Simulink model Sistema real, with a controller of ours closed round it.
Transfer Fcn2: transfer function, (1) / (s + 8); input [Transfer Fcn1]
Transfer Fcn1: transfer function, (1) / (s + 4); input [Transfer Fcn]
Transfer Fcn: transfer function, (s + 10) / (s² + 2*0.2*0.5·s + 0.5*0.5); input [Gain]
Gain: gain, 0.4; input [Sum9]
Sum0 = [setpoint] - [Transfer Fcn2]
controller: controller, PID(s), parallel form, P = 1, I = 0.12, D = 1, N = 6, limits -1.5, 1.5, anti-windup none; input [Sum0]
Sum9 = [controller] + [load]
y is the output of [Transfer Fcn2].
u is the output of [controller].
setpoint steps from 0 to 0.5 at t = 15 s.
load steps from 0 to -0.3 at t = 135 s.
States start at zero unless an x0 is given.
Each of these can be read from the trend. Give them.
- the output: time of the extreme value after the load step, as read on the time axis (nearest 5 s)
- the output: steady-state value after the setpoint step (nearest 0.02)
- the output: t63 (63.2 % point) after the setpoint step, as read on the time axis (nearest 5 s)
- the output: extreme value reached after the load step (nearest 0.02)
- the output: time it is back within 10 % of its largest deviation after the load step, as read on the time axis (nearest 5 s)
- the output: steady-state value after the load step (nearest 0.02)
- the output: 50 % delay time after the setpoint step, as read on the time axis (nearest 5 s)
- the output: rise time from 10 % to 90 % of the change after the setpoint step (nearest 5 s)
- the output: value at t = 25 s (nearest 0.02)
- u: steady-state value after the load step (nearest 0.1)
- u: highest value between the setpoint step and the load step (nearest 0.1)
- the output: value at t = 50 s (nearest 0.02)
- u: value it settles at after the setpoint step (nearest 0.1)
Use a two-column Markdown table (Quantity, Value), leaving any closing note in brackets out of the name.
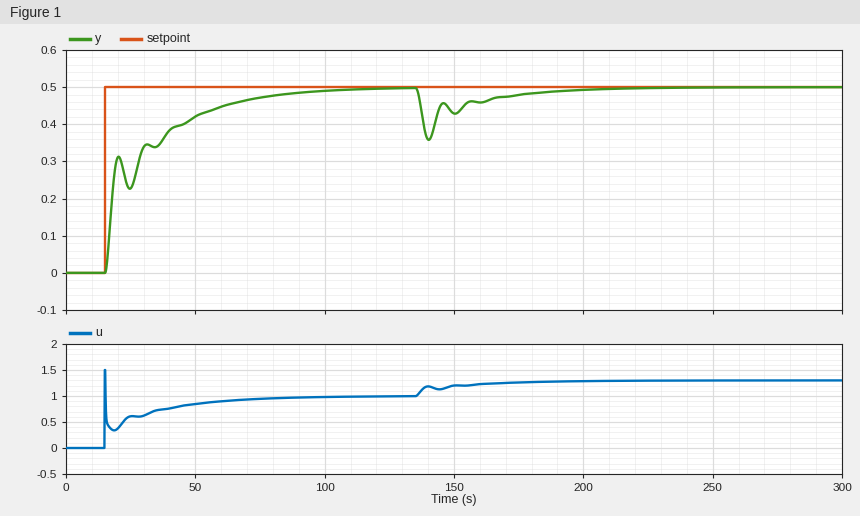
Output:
| Quantity | Value |
|---|---|
| the output: time of the extreme value after the load step, as read on the time axis | 140 s |
| the output: steady-state value after the setpoint step | 0.50 |
| the output: t63 (63.2 % point) after the setpoint step, as read on the time axis | 30 s |
| the output: extreme value reached after the load step | 0.36 |
| the output: time it is back within 10 % of its largest deviation after the load step, as read on the time axis | 185 s |
| the output: steady-state value after the load step | 0.50 |
| the output: 50 % delay time after the setpoint step, as read on the time axis | 20 s |
| the output: rise time from 10 % to 90 % of the change after the setpoint step | 45 s |
| the output: value at t = 25 s | 0.22 |
| u: steady-state value after the load step | 1.3 |
| u: highest value between the setpoint step and the load step | 1.5 |
| the output: value at t = 50 s | 0.42 |
| u: value it settles at after the setpoint step | 1.0 |
